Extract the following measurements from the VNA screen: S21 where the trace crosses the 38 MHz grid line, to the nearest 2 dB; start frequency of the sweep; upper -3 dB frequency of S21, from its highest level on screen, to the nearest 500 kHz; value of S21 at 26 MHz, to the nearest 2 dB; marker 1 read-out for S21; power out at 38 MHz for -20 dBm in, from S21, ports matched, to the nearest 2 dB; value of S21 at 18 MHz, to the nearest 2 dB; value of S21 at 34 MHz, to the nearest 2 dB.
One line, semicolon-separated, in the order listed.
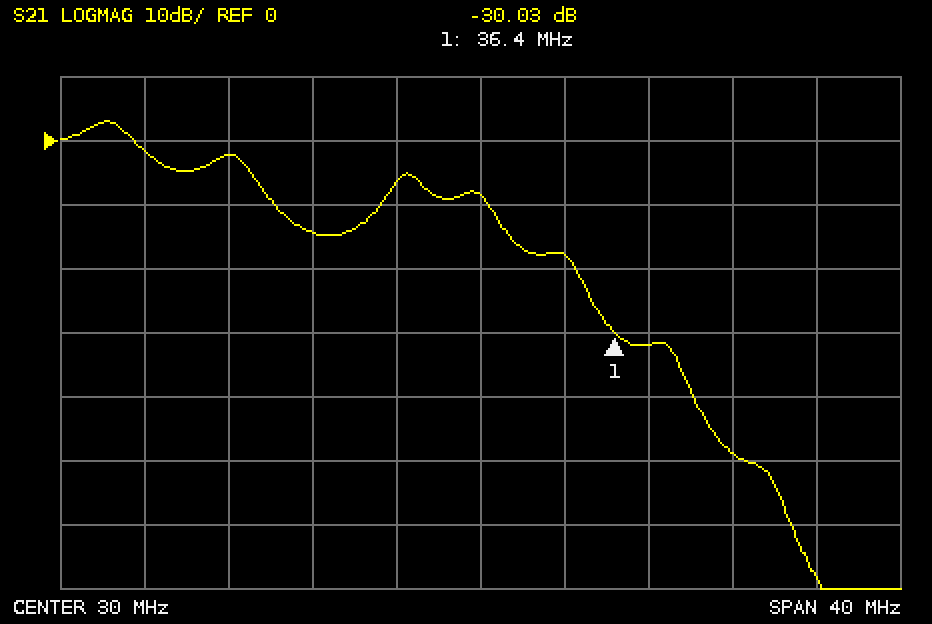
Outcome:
-32 dB; 10 MHz; 13.5 MHz; -6 dB; -30.03 dB; -52 dBm; -2 dB; -18 dB
